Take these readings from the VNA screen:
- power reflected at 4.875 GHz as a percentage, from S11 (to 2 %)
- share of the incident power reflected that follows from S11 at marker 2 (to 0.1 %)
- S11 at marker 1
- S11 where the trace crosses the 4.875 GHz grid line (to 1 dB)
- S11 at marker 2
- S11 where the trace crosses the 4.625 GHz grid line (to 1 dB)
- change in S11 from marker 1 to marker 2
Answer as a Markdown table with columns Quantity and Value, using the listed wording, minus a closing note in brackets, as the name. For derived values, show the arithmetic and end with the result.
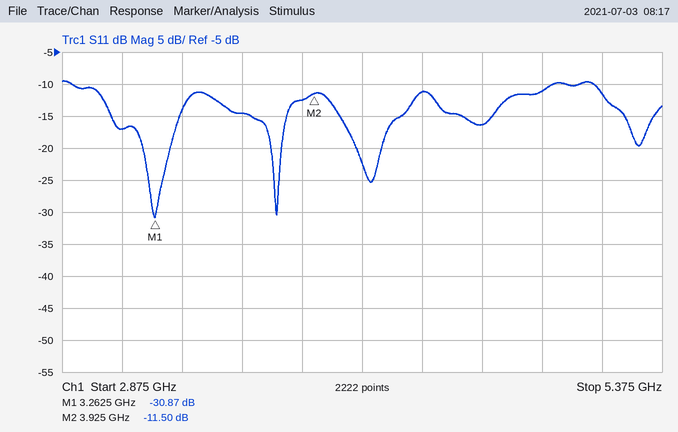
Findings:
| Quantity | Value |
|---|---|
| power reflected at 4.875 GHz as a percentage, from S11 | 10^(-11/10) ≈ 8 % |
| share of the incident power reflected that follows from S11 at marker 2 | 10^(-11.5/10) ≈ 7.1 % |
| S11 at marker 1 | -30.87 dB |
| S11 where the trace crosses the 4.875 GHz grid line | -11 dB |
| S11 at marker 2 | -11.50 dB |
| S11 where the trace crosses the 4.625 GHz grid line | -16 dB |
| change in S11 from marker 1 to marker 2 | -11.5 − (-30.87) = 19.37 dB |
